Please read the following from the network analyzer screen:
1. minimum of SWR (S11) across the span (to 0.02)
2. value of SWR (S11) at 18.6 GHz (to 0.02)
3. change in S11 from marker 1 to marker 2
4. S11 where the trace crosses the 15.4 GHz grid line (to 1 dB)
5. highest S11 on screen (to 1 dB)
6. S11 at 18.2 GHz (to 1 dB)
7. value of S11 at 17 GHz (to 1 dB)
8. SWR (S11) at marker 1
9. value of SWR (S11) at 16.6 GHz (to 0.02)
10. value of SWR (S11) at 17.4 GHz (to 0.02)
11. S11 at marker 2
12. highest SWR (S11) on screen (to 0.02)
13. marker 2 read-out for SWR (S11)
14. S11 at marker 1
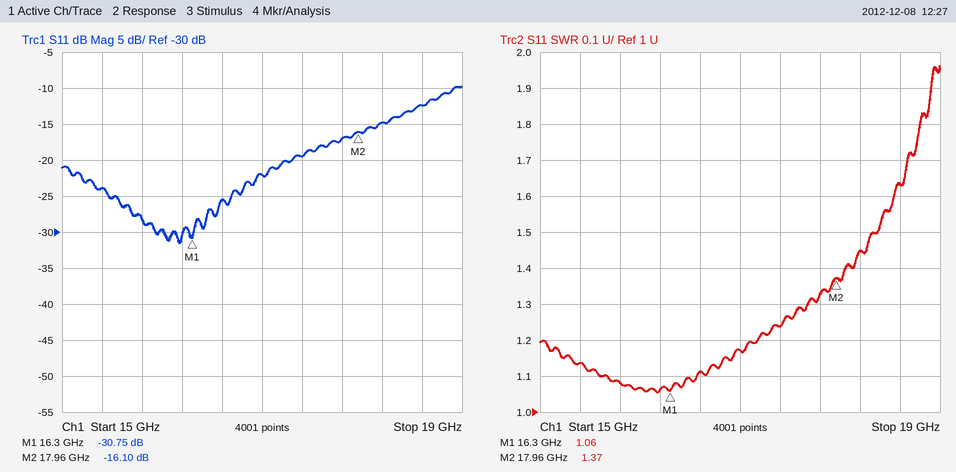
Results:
1.06
1.64
14.65 dB
-24 dB
-10 dB
-15 dB
-22 dB
1.06
1.12
1.24
-16.10 dB
1.96
1.37
-30.75 dB
